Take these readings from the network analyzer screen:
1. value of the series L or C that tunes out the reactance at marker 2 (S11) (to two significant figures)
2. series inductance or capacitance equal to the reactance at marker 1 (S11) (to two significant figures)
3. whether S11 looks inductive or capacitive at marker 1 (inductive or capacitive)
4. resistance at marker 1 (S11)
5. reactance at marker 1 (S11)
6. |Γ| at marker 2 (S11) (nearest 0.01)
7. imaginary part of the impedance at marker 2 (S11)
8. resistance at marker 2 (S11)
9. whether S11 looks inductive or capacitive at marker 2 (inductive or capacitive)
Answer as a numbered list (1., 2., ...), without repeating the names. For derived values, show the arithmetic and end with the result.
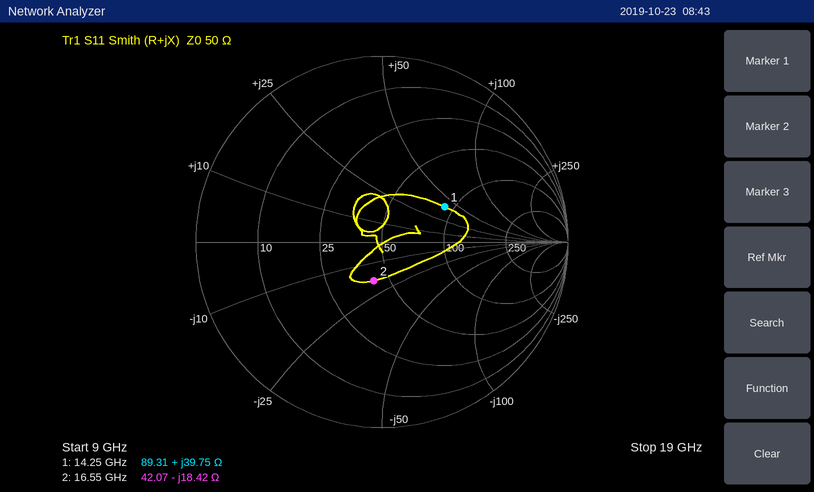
1. L = 18.42 Ω/(2π × 16.55 GHz) ≈ 177 pH, so 180 pH to two significant figures
2. L = 39.75 Ω/(2π × 14.25 GHz) ≈ 444 pH, so 440 pH to two significant figures
3. inductive
4. 89.31 Ω
5. +39.75 Ω
6. 0.21
7. -18.42 Ω
8. 42.07 Ω
9. capacitive
